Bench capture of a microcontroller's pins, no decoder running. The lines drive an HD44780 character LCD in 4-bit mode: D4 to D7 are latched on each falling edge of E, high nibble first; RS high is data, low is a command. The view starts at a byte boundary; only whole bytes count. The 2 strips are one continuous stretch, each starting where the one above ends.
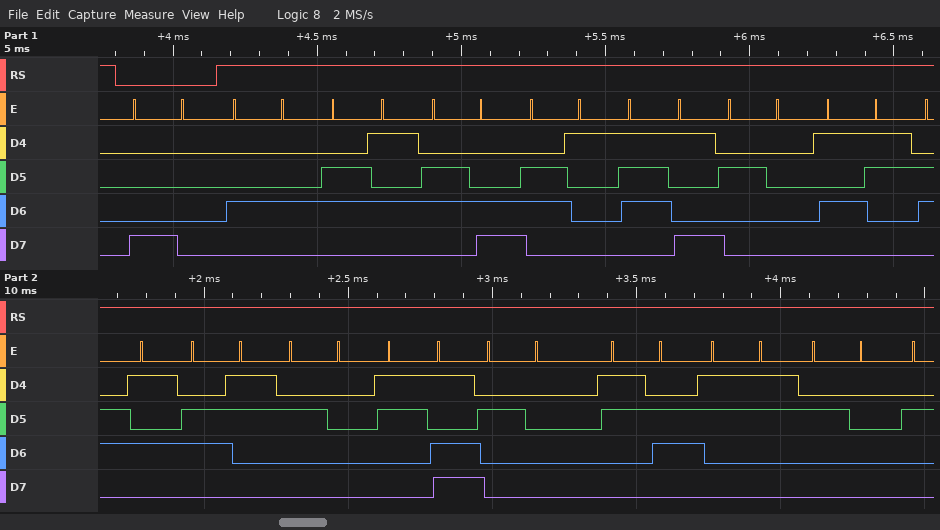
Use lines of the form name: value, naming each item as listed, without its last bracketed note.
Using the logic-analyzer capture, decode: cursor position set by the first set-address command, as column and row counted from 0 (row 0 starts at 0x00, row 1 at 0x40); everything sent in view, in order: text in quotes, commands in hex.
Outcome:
cursor position set by the first set-address command, as column and row counted from 0: column 0, row 0
everything sent in view, in order: text in quotes, commands in hex: 0x80 "Delay Sec = 63 "
